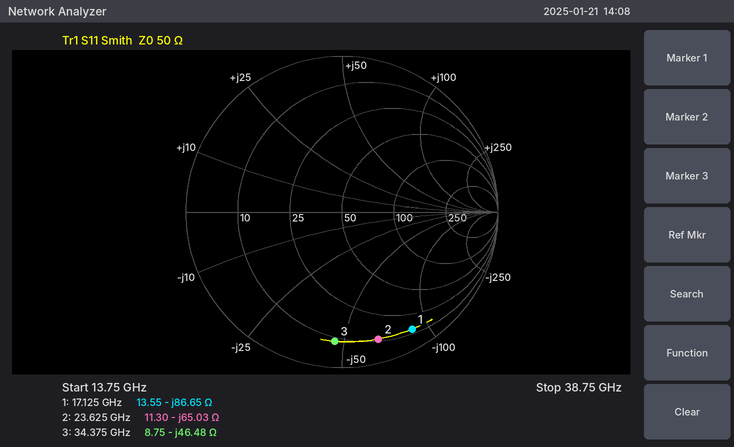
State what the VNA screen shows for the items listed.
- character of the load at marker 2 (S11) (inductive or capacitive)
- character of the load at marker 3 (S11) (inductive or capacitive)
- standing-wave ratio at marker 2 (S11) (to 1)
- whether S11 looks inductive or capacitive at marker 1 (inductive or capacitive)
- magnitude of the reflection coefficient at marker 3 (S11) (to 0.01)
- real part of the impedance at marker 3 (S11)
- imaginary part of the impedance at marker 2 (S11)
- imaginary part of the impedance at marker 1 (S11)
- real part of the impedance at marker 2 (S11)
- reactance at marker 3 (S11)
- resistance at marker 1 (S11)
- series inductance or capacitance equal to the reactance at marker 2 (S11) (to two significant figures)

capacitive
capacitive
12
capacitive
0.83
8.75 Ω
-65.03 Ω
-86.65 Ω
11.30 Ω
-46.48 Ω
13.55 Ω
100 fF
